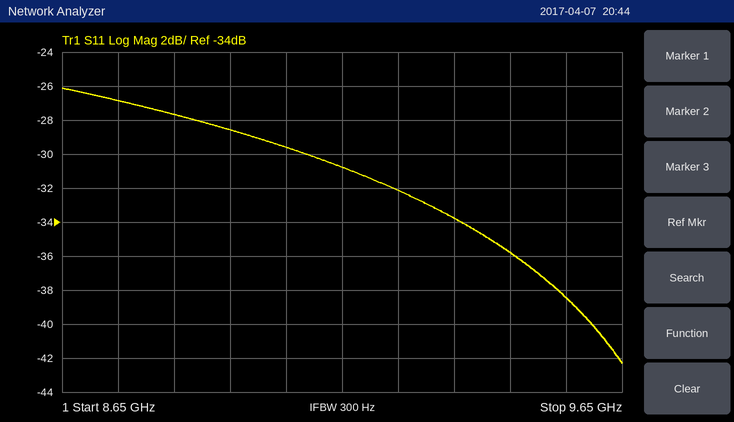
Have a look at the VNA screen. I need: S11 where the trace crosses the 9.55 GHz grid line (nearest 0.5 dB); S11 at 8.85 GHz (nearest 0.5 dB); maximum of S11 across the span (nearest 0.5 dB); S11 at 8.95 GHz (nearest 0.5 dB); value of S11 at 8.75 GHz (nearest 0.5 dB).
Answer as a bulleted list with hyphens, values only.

- -38.5 dB
- -27.5 dB
- -26.0 dB
- -28.5 dB
- -27.0 dB
